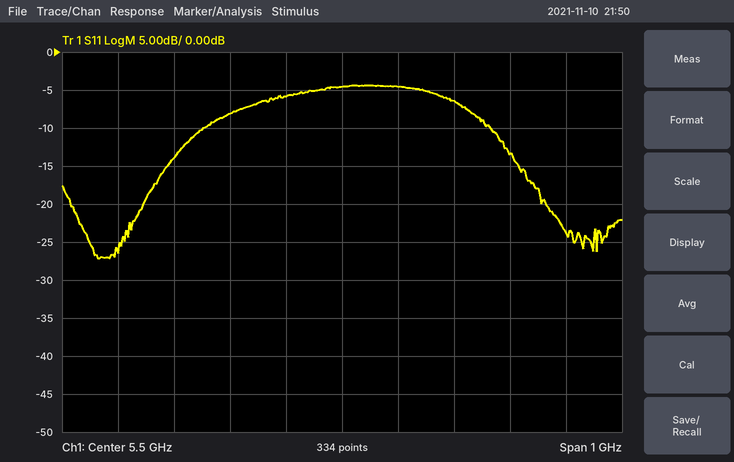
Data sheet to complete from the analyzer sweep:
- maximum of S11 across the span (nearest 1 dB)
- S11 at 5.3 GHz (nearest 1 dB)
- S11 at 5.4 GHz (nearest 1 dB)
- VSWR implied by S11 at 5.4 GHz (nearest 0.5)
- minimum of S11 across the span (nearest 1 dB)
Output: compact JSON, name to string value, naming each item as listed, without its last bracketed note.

{"maximum of S11 across the span": "-4 dB", "S11 at 5.3 GHz": "-8 dB", "S11 at 5.4 GHz": "-6 dB", "VSWR implied by S11 at 5.4 GHz": "3.0", "minimum of S11 across the span": "-27 dB"}
